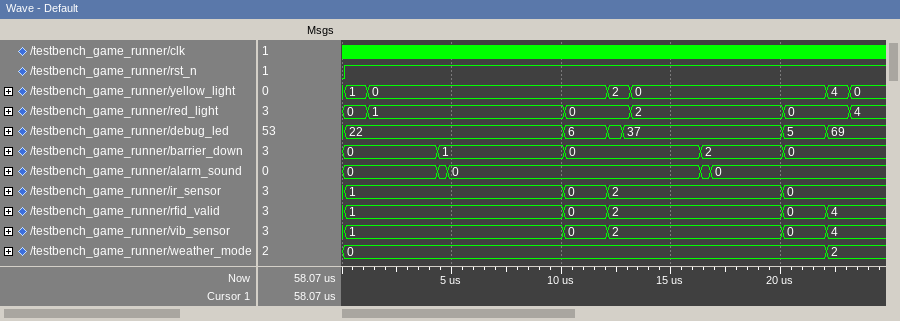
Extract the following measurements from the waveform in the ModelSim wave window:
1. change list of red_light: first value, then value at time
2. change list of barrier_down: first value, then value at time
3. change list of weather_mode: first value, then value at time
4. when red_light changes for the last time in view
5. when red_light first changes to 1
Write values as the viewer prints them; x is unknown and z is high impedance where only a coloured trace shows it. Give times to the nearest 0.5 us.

0, 1 at 1 us, 0 at 10 us, 2 at 13 us, 0 at 20 us, 4 at 23 us
0, 1 at 4.5 us, 0 at 10 us, 2 at 16.5 us, 0 at 20 us
0, 2 at 22 us
23 us
1 us
